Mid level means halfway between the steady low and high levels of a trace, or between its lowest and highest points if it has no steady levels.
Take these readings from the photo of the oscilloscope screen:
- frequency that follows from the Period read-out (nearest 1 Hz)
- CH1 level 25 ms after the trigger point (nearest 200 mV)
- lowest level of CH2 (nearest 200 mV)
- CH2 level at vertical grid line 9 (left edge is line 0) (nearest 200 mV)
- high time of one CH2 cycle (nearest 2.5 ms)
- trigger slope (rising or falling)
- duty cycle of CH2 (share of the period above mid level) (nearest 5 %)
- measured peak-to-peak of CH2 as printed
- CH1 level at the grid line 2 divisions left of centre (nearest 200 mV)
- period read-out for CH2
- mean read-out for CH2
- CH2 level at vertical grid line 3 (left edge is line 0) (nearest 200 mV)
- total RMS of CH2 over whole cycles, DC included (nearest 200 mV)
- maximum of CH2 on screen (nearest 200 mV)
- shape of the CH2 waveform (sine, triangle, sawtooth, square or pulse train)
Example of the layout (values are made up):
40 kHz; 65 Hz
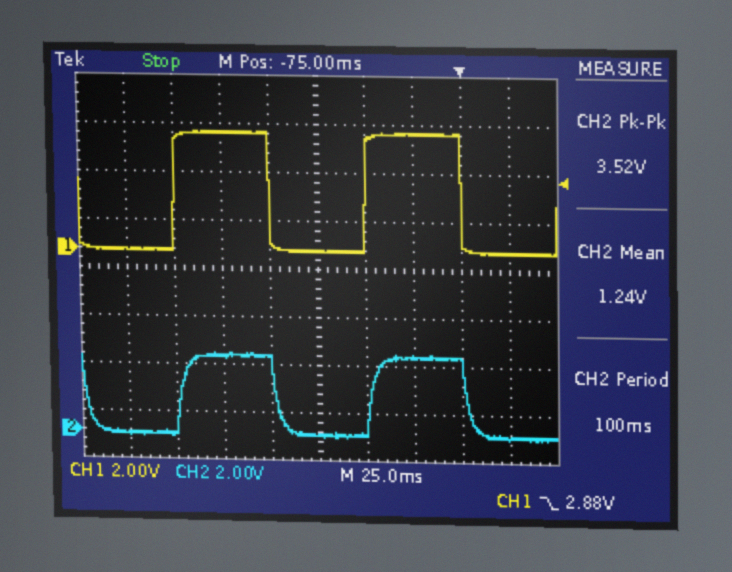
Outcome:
10 Hz; 0.0 V; -200 mV; -200 mV; 50.0 ms; falling; 50 %; 3.52 V; 4.8 V; 100 ms; 1.24 V; 3.2 V; 2.2 V; 3.2 V; square
